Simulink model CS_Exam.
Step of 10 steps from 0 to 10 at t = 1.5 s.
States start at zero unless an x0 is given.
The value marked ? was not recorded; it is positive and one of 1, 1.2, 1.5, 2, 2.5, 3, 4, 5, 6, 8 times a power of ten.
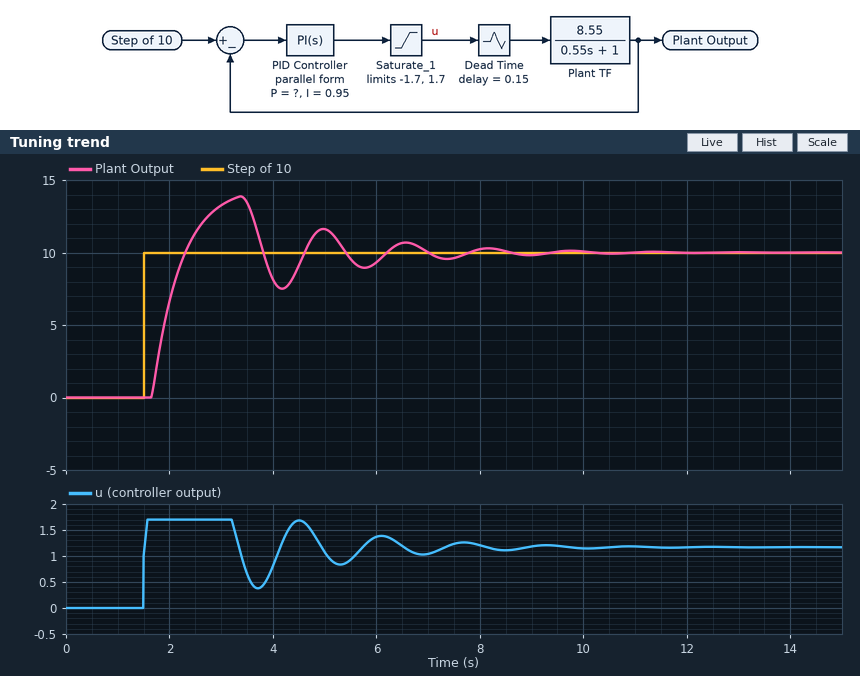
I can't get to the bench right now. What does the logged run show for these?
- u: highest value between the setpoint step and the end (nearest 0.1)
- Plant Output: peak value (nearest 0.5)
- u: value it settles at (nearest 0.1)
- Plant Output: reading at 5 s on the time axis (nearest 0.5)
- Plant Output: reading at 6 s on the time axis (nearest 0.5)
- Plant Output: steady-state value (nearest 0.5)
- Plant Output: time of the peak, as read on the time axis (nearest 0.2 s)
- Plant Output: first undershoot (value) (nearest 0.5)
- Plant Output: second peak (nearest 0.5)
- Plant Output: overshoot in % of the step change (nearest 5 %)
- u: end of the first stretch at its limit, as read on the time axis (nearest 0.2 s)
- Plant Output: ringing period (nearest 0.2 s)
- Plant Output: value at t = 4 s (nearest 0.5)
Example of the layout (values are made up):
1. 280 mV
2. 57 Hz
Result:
1. 1.7
2. 14.0
3. 1.2
4. 11.5
5. 9.5
6. 10.0
7. 3.4 s
8. 7.5
9. 11.5
10. 40 %
11. 3.2 s
12. 1.6 s
13. 8.0
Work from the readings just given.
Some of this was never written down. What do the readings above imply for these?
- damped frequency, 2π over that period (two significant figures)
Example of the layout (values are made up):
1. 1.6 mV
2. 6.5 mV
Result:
1. 3.9 rad/s
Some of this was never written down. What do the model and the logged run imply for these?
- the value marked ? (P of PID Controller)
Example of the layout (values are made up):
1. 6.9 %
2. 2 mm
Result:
1. 0.1
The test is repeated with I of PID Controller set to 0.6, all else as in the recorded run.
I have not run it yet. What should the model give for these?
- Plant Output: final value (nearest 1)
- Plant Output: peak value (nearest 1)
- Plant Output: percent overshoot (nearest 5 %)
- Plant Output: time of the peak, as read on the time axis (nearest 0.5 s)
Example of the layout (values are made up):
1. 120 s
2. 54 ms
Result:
1. 10
2. 13
3. 35 %
4. 3.0 s
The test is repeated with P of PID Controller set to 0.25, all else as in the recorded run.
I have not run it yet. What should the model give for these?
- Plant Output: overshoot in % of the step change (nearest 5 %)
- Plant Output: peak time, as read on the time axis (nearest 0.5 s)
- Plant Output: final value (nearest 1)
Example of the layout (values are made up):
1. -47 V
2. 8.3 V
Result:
1. 35 %
2. 3.0 s
3. 10
